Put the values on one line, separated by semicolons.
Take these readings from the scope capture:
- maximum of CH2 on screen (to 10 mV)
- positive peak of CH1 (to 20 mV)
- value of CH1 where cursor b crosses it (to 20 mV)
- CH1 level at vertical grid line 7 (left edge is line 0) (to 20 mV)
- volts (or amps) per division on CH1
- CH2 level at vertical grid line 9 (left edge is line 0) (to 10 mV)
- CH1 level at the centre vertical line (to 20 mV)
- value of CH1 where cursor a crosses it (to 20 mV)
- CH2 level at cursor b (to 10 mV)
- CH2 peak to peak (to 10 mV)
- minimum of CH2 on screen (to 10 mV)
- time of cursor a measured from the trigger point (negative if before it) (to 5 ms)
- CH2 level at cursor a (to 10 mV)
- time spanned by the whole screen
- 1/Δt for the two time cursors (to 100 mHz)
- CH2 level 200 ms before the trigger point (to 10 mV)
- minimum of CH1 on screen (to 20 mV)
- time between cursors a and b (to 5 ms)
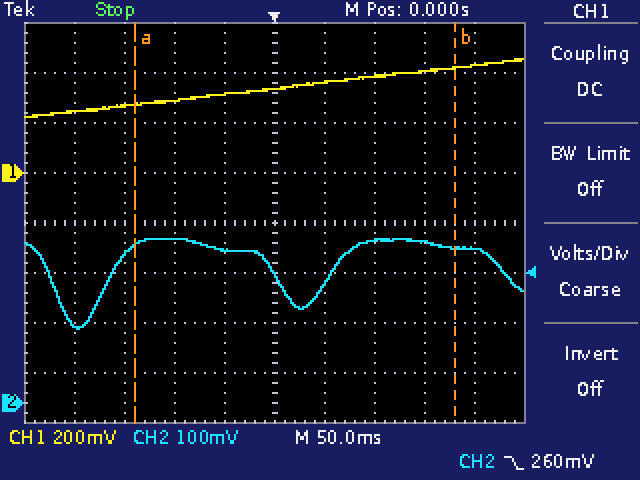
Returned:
330 mV; 460 mV; 420 mV; 380 mV; 200 mV; 310 mV; 340 mV; 280 mV; 310 mV; 180 mV; 150 mV; -140 ms; 310 mV; 500 ms; 3.1 Hz; 160 mV; 220 mV; 320 ms
